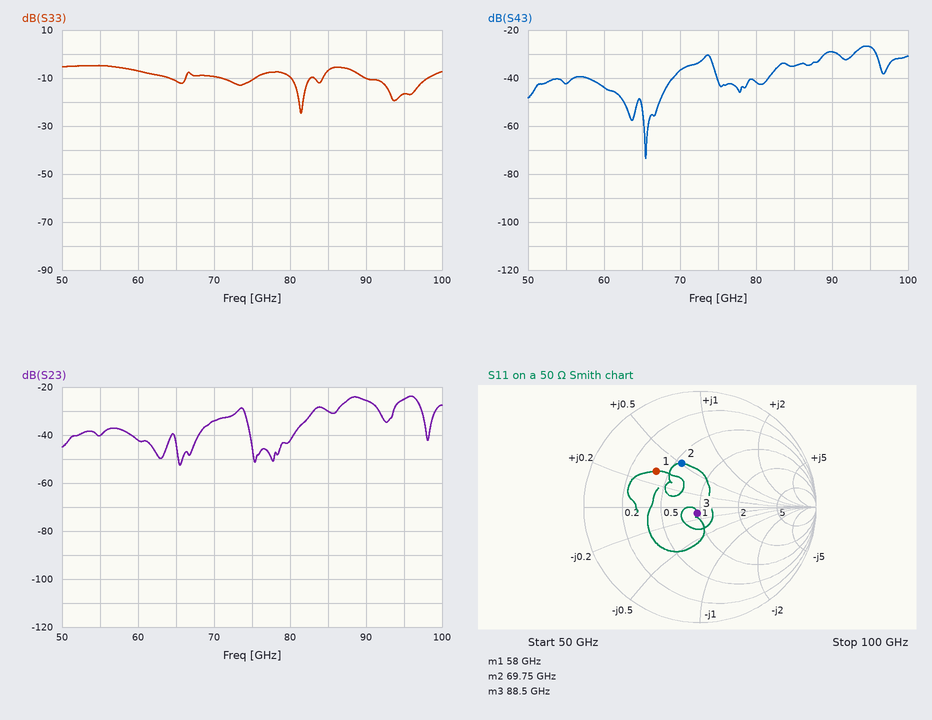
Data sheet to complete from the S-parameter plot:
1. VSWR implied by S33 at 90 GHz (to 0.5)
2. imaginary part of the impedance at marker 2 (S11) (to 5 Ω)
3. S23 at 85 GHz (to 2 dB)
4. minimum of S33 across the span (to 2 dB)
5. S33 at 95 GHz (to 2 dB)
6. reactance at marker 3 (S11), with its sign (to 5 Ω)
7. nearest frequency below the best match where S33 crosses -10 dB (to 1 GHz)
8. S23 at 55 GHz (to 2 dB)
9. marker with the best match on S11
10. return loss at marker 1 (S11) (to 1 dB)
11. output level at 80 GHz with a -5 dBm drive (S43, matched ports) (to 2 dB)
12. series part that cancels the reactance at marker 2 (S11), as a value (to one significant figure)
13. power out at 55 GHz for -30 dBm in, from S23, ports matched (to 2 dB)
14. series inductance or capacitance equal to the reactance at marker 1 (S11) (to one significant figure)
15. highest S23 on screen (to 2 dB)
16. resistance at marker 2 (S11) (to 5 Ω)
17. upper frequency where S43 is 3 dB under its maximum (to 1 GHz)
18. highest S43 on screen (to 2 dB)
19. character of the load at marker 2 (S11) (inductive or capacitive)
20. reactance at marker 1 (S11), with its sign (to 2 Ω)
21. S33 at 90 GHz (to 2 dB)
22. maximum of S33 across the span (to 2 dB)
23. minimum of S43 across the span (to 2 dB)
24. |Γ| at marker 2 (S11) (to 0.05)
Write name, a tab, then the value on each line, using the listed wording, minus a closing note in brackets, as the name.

VSWR implied by S33 at 90 GHz	2.0
imaginary part of the impedance at marker 2 (S11)	+25 Ω
S23 at 85 GHz	-30 dB
minimum of S33 across the span	-24 dB
S33 at 95 GHz	-16 dB
reactance at marker 3 (S11), with its sign	-5 Ω
nearest frequency below the best match where S33 crosses -10 dB	80 GHz
S23 at 55 GHz	-40 dB
marker with the best match on S11	marker 3
return loss at marker 1 (S11)	6 dB
output level at 80 GHz with a -5 dBm drive (S43, matched ports)	-46 dBm
series part that cancels the reactance at marker 2 (S11), as a value	90 fF
power out at 55 GHz for -30 dBm in, from S23, ports matched	-70 dBm
series inductance or capacitance equal to the reactance at marker 1 (S11)	40 pH
highest S23 on screen	-24 dB
resistance at marker 2 (S11)	30 Ω
upper frequency where S43 is 3 dB under its maximum	96 GHz
highest S43 on screen	-26 dB
character of the load at marker 2 (S11)	inductive
reactance at marker 1 (S11), with its sign	+16 Ω
S33 at 90 GHz	-10 dB
maximum of S33 across the span	-4 dB
minimum of S43 across the span	-74 dB
|Γ| at marker 2 (S11)	0.40
